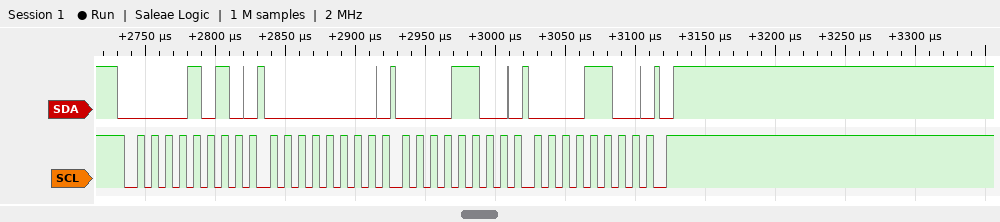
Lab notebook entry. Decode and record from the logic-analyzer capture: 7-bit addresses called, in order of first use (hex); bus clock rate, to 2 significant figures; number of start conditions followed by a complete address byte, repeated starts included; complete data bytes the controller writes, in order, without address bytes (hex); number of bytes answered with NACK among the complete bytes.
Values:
0x05
100 kHz
1
00 0C 0C
0
